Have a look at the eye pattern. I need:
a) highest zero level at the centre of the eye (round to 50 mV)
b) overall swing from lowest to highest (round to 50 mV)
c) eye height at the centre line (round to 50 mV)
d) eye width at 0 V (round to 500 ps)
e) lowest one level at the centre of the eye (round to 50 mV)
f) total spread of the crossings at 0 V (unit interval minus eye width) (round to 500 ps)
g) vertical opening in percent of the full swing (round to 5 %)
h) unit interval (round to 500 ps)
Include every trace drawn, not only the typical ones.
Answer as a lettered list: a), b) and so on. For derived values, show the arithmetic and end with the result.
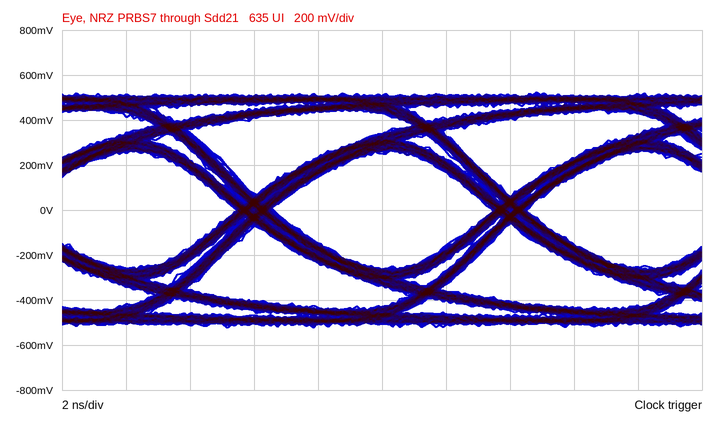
a) -250 mV
b) 1.05 V
c) 500 mV
d) 7.0 ns
e) 250 mV
f) 1.0 ns
g) 500 mV / 1.05 V ≈ 47.6 %, so 50 % to the nearest 5 %
h) 8.0 ns
